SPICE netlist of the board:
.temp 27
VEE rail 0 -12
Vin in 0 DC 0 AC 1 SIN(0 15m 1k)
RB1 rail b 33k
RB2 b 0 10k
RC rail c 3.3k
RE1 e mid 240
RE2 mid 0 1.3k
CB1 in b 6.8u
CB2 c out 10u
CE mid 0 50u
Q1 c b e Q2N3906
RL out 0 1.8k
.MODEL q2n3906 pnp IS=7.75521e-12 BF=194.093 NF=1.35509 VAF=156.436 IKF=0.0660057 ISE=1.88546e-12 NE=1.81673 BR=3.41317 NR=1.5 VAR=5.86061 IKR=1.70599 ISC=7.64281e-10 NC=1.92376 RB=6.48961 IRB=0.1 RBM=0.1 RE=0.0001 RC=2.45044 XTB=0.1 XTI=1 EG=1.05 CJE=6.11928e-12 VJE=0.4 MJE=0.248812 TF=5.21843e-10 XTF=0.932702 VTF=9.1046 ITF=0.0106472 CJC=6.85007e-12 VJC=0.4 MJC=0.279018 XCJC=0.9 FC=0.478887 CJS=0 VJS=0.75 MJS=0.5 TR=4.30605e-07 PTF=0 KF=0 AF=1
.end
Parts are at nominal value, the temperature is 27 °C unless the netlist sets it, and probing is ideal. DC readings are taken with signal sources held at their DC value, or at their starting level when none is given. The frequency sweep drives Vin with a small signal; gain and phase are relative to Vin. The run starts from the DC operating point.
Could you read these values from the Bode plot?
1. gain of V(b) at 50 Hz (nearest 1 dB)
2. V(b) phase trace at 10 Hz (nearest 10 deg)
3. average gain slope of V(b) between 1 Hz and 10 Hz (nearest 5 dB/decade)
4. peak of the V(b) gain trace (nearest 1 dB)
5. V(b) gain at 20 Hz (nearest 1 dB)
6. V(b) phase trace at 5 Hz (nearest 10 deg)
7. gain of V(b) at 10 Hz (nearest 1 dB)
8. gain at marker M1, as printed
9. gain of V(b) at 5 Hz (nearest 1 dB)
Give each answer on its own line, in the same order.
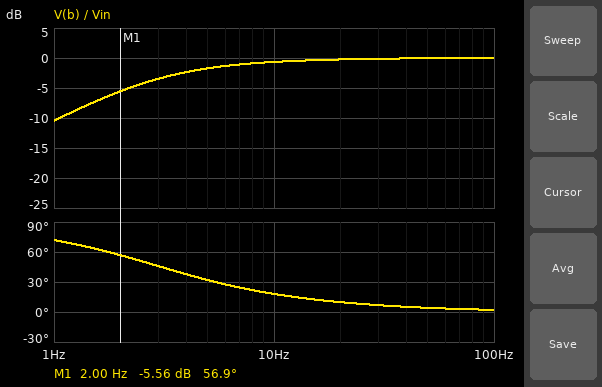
0 dB
20 deg
10 dB/decade
0 dB
0 dB
30 deg
-1 dB
-5.56 dB
-2 dB
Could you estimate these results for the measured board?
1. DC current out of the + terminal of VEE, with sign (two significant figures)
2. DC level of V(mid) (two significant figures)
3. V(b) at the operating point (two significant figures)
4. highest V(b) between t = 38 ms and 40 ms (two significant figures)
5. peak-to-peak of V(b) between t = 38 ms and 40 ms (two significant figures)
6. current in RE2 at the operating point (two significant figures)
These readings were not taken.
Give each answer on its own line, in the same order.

-1.6 mA
-1.7 V
-2.7 V
-2.7 V
30 mV
1.3 mA
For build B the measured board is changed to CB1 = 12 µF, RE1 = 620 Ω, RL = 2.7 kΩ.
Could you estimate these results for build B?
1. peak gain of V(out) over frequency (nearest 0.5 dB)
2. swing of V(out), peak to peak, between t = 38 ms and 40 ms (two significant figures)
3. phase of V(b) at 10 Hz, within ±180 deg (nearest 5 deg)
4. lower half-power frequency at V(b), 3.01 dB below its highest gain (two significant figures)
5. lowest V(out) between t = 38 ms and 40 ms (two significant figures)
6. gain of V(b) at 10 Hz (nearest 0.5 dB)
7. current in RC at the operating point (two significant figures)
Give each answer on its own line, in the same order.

7.0 dB
68 mV
10 deg
1.8 Hz
-34 mV
0 dB
1.1 mA
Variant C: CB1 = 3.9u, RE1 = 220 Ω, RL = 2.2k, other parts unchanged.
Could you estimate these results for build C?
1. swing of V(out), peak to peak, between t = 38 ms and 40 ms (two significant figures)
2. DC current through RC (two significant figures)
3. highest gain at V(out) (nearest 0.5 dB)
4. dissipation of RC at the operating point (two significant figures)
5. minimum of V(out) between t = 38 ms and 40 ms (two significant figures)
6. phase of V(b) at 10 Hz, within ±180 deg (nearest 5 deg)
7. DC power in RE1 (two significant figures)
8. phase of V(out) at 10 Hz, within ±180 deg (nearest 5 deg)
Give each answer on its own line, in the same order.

160 mV
1.3 mA
14.5 dB
5.9 mW
-79 mV
30 deg
400 µW
-90 deg
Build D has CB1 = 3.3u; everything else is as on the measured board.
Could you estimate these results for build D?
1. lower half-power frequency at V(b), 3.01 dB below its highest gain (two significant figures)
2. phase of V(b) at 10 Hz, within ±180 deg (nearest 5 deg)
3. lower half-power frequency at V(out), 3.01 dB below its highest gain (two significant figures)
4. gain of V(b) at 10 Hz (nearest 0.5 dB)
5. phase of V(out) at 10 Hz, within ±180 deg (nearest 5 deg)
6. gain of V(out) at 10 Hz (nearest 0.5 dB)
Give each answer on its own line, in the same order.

7.2 Hz
35 deg
18 Hz
-2.0 dB
-90 deg
5.5 dB
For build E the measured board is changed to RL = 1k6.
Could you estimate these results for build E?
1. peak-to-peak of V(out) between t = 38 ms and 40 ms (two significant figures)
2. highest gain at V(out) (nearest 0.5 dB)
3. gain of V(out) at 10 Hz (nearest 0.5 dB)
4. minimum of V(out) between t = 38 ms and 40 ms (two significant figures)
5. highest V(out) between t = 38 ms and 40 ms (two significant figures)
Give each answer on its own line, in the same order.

120 mV
12.0 dB
6.5 dB
-60 mV
60 mV
